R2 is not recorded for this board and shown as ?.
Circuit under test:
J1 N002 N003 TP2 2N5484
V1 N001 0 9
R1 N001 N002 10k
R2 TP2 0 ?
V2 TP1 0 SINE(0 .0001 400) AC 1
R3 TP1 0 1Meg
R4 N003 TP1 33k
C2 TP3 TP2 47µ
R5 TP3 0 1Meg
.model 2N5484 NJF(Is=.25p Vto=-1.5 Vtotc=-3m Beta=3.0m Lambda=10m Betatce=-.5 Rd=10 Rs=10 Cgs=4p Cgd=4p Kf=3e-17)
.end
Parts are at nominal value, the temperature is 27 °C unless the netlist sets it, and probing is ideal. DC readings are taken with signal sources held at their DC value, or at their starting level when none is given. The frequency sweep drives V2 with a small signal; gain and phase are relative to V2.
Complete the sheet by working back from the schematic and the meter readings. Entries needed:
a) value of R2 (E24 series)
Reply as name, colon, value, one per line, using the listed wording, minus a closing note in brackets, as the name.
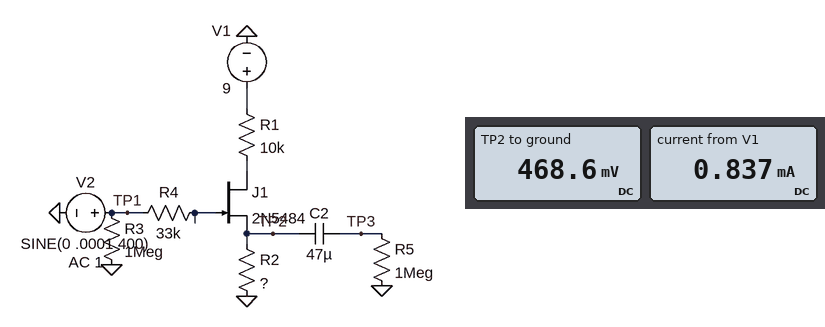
value of R2: 560 Ω
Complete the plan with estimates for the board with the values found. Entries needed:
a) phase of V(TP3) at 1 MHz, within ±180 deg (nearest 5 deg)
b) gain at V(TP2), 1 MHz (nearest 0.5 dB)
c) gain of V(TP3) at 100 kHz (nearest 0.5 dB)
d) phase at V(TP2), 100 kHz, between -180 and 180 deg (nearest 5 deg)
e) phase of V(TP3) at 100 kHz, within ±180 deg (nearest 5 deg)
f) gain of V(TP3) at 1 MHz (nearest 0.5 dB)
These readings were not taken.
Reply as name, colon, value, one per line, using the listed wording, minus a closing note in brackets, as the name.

phase of V(TP3) at 1 MHz, within ±180 deg: 15 deg
gain at V(TP2), 1 MHz: -37.0 dB
gain of V(TP3) at 100 kHz: -41.0 dB
phase at V(TP2), 100 kHz, between -180 and 180 deg: 5 deg
phase of V(TP3) at 100 kHz, within ±180 deg: 5 deg
gain of V(TP3) at 1 MHz: -37.0 dB
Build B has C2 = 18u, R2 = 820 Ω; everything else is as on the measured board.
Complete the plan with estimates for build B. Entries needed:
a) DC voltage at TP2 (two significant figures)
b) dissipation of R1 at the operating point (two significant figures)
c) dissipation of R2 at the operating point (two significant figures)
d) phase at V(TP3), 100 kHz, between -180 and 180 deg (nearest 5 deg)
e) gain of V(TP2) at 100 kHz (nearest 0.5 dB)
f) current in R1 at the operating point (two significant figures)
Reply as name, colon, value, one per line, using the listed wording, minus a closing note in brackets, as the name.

DC voltage at TP2: 670 mV
dissipation of R1 at the operating point: 6.6 mW
dissipation of R2 at the operating point: 540 µW
phase at V(TP3), 100 kHz, between -180 and 180 deg: 0 deg
gain of V(TP2) at 100 kHz: -33.5 dB
current in R1 at the operating point: 810 µA
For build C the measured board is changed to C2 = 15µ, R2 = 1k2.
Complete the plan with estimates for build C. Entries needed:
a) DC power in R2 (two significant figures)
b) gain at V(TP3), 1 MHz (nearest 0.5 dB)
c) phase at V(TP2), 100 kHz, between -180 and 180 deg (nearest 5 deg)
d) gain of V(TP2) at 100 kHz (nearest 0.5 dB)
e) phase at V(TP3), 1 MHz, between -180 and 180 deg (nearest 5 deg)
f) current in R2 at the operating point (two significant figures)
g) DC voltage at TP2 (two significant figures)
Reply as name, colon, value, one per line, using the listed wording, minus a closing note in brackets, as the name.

DC power in R2: 720 µW
gain at V(TP3), 1 MHz: -24.0 dB
phase at V(TP2), 100 kHz, between -180 and 180 deg: -5 deg
gain of V(TP2) at 100 kHz: -19.0 dB
phase at V(TP3), 1 MHz, between -180 and 180 deg: -35 deg
current in R2 at the operating point: 770 µA
DC voltage at TP2: 930 mV
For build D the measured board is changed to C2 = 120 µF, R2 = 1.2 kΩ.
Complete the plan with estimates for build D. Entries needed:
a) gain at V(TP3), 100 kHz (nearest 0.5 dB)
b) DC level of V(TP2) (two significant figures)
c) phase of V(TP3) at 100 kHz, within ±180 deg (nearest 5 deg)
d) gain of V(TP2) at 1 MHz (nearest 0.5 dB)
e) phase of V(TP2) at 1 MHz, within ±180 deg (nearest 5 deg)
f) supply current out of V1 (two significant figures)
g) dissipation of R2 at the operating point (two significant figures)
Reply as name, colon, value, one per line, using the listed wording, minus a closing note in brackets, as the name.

gain at V(TP3), 100 kHz: -19.0 dB
DC level of V(TP2): 930 mV
phase of V(TP3) at 100 kHz, within ±180 deg: -5 deg
gain of V(TP2) at 1 MHz: -24.0 dB
phase of V(TP2) at 1 MHz, within ±180 deg: -35 deg
supply current out of V1: 770 µA
dissipation of R2 at the operating point: 720 µW
